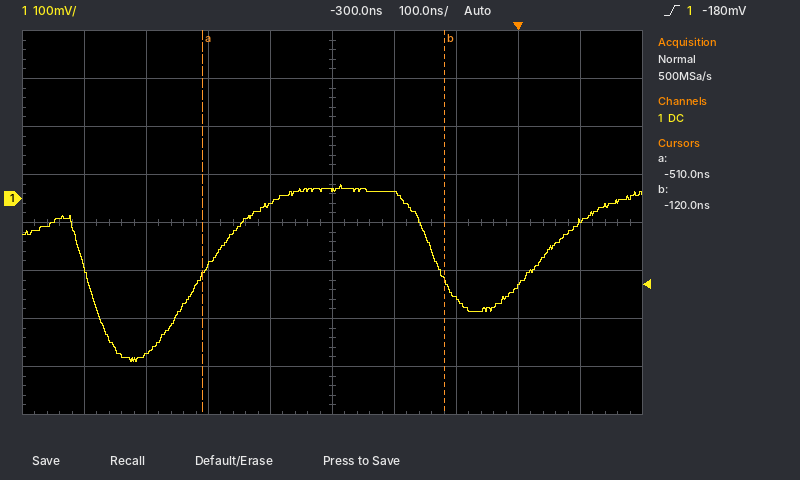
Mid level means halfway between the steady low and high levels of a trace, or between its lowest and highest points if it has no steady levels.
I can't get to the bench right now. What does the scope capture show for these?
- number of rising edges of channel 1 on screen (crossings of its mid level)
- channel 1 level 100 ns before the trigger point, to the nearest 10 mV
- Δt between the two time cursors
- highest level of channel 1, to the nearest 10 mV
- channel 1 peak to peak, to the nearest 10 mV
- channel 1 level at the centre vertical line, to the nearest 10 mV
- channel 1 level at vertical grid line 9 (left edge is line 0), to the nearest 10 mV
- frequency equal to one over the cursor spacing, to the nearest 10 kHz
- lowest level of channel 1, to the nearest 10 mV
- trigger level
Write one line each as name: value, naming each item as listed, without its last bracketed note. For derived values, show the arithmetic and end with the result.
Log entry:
number of rising edges of channel 1 on screen: 2
channel 1 level 100 ns before the trigger point, to the nearest 10 mV: -210 mV
Δt between the two time cursors: -120 ns − (-510 ns) = 390 ns
highest level of channel 1, to the nearest 10 mV: 30 mV
channel 1 peak to peak, to the nearest 10 mV: 30 mV − (-340 mV) = 370 mV
channel 1 level at the centre vertical line, to the nearest 10 mV: 20 mV
channel 1 level at vertical grid line 9 (left edge is line 0), to the nearest 10 mV: -50 mV
frequency equal to one over the cursor spacing, to the nearest 10 kHz: 1 / 390 ns ≈ 2.56 MHz
lowest level of channel 1, to the nearest 10 mV: -340 mV
trigger level: -180 mV
